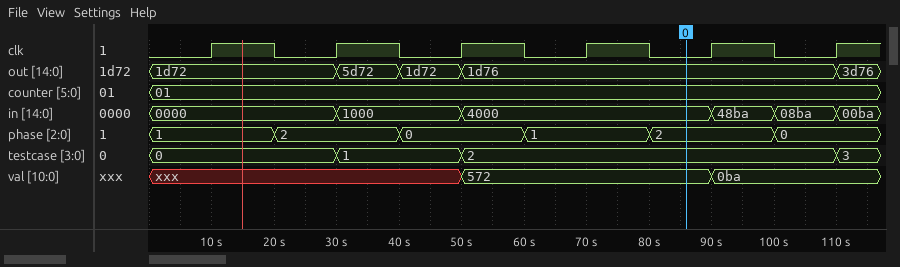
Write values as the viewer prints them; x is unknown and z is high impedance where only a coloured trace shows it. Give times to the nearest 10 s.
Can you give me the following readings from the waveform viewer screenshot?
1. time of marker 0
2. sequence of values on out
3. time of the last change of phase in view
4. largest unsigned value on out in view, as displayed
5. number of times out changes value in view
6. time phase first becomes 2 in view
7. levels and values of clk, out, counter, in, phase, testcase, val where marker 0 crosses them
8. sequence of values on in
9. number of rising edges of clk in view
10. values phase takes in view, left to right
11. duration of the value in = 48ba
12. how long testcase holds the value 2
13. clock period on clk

90 s
1d72, 5d72, 1d72, 1d76, 3d76
100 s
5d72
4
20 s
clk=0, out=1d76, counter=01, in=4000, phase=2, testcase=2, val=572
0000, 1000, 4000, 48ba, 08ba, 00ba
6
1, 2, 0, 1, 2, 0
10 s
60 s
20 s
